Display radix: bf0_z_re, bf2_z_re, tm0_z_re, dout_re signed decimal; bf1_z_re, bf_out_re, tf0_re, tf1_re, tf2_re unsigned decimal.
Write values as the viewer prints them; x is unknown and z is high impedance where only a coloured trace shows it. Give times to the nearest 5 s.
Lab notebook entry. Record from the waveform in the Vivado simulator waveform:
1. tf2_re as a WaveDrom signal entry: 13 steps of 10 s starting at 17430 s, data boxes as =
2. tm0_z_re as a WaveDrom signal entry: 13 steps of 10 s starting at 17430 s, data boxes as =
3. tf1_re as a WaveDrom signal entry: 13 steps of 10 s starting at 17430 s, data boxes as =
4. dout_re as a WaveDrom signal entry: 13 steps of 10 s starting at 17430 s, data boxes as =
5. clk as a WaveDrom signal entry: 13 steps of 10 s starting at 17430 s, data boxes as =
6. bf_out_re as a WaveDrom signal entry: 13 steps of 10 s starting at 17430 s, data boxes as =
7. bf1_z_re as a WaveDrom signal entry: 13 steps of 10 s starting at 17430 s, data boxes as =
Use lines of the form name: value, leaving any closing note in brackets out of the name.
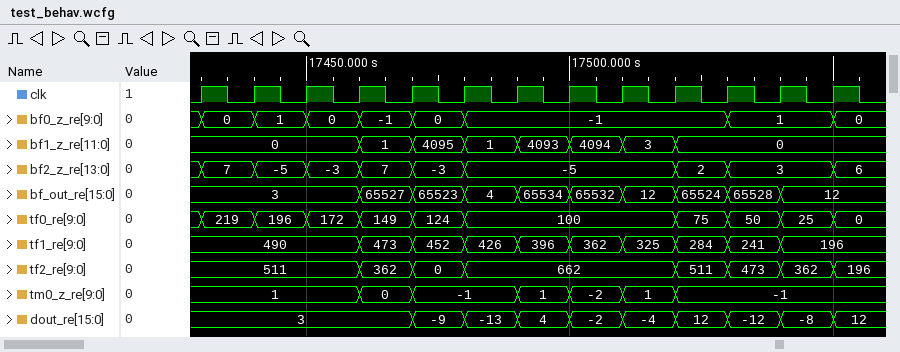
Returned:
tf2_re as a WaveDrom signal entry: 13 steps of 10 s starting at 17430 s, data boxes as =: {name: 'tf2_re', wave: '=..===...====', data: '511 362 0 662 511 473 362 196'}
tm0_z_re as a WaveDrom signal entry: 13 steps of 10 s starting at 17430 s, data boxes as =: {name: 'tm0_z_re', wave: '=..==.====...', data: '1 0 -1 1 -2 1 -1'}
tf1_re as a WaveDrom signal entry: 13 steps of 10 s starting at 17430 s, data boxes as =: {name: 'tf1_re', wave: '=..=========.', data: '490 473 452 426 396 362 325 284 241 196'}
dout_re as a WaveDrom signal entry: 13 steps of 10 s starting at 17430 s, data boxes as =: {name: 'dout_re', wave: '=...=========', data: '3 -9 -13 4 -2 -4 12 -12 -8 12'}
clk as a WaveDrom signal entry: 13 steps of 10 s starting at 17430 s, data boxes as =: {name: 'clk', wave: 'p............'}
bf_out_re as a WaveDrom signal entry: 13 steps of 10 s starting at 17430 s, data boxes as =: {name: 'bf_out_re', wave: '=..=========.', data: '3 65527 65523 4 65534 65532 12 65524 65528 12'}
bf1_z_re as a WaveDrom signal entry: 13 steps of 10 s starting at 17430 s, data boxes as =: {name: 'bf1_z_re', wave: '=..=======...', data: '0 1 4095 1 4093 4094 3 0'}
